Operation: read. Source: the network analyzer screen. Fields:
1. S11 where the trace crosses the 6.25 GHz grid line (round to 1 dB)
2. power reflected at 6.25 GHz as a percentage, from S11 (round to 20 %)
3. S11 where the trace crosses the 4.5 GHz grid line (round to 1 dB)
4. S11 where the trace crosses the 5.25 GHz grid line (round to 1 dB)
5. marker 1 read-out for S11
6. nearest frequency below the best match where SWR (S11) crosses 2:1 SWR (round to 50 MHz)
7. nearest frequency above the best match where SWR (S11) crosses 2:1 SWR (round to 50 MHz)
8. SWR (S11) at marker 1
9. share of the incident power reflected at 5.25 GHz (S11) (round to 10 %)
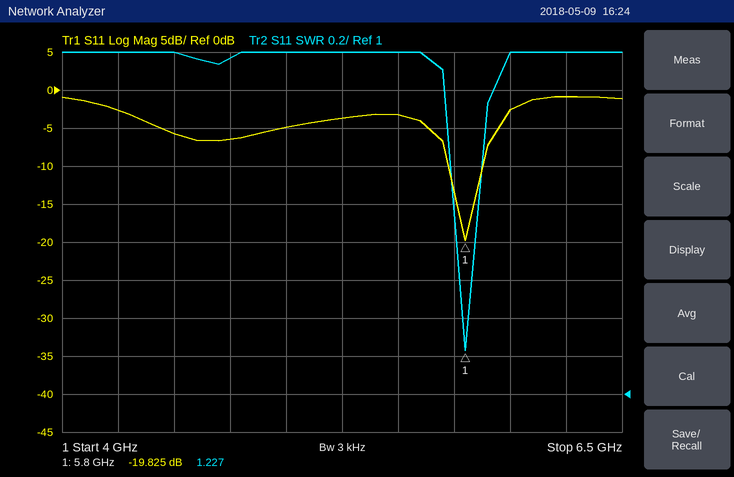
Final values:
-1 dB
80 %
-6 dB
-4 dB
-19.825 dB
5.75 GHz
5.85 GHz
1.227
40 %
